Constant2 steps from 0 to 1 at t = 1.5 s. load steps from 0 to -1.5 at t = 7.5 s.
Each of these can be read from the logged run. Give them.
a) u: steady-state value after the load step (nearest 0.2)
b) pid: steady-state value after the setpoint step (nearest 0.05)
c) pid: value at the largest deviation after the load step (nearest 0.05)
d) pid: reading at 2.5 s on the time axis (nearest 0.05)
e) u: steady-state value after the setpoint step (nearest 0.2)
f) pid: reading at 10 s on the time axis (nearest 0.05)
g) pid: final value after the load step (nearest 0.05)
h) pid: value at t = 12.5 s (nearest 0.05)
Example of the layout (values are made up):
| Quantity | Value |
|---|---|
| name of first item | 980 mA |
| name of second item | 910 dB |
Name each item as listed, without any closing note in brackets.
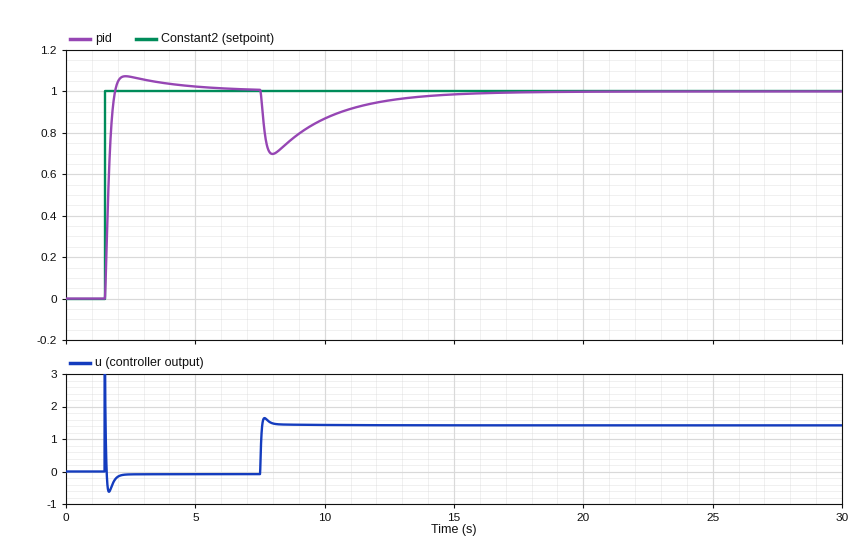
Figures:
| Quantity | Value |
|---|---|
| u: steady-state value after the load step | 1.4 |
| pid: steady-state value after the setpoint step | 1.00 |
| pid: value at the largest deviation after the load step | 0.70 |
| pid: reading at 2.5 s on the time axis | 1.05 |
| u: steady-state value after the setpoint step | 0.0 |
| pid: reading at 10 s on the time axis | 0.85 |
| pid: final value after the load step | 1.00 |
| pid: value at t = 12.5 s | 0.95 |
